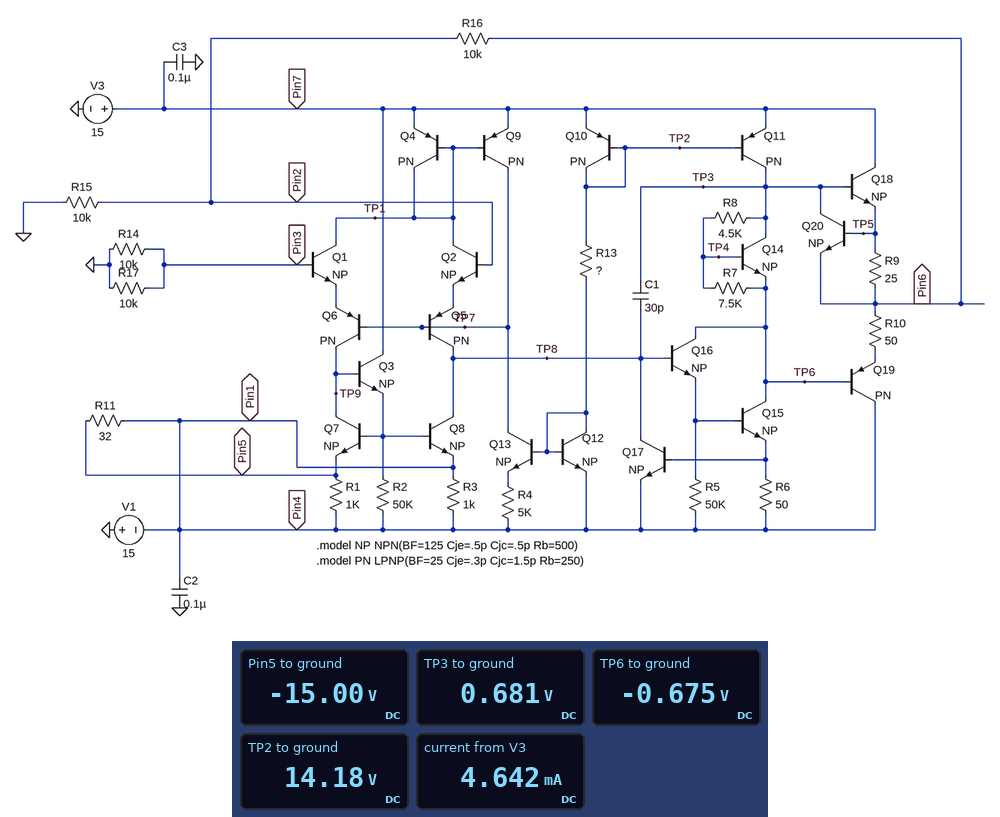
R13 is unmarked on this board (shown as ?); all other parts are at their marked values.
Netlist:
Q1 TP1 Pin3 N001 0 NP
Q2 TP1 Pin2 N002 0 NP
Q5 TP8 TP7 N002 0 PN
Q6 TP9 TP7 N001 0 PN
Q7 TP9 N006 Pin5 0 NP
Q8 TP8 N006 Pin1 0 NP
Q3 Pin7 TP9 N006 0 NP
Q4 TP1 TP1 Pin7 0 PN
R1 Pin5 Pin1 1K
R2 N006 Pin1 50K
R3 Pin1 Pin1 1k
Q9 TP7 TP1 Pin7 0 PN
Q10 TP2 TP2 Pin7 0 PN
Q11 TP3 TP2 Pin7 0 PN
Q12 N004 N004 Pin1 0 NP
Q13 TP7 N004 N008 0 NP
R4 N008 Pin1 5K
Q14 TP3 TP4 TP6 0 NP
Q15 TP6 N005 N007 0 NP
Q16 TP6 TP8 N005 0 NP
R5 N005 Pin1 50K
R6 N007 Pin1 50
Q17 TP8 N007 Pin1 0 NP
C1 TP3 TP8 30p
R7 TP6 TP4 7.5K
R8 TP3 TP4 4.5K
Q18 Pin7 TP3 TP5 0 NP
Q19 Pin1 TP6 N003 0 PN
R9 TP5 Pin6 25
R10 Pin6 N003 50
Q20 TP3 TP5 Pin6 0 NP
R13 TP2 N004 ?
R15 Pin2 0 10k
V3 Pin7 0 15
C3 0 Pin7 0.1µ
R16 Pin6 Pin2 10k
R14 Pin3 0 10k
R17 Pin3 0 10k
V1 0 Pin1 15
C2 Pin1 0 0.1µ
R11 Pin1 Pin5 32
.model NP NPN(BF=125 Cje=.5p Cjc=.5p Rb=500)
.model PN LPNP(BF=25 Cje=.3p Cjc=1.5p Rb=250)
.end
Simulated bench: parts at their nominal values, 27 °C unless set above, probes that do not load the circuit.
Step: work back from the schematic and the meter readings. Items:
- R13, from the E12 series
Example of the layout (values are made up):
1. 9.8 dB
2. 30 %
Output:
1. 12 kΩ
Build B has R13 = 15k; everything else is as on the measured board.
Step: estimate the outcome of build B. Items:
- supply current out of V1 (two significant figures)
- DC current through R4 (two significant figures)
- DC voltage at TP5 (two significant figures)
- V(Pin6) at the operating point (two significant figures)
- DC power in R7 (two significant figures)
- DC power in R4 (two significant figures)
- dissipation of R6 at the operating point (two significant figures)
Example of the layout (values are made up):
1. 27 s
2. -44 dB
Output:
1. 3.7 mA
2. 24 µA
3. 3.1 mV
4. 2.7 mV
5. 84 µW
6. 2.9 µW
7. 150 µW
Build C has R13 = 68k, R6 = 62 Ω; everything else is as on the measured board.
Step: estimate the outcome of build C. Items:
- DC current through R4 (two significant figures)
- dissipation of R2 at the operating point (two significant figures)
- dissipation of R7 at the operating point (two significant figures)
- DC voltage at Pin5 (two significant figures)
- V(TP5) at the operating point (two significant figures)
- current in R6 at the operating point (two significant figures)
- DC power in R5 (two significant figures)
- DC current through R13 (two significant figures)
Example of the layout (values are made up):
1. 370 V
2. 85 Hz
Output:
1. 17 µA
2. 8.5 µW
3. 74 µW
4. -15 V
5. 1.6 mV
6. 370 µA
7. 12 µW
8. 420 µA
